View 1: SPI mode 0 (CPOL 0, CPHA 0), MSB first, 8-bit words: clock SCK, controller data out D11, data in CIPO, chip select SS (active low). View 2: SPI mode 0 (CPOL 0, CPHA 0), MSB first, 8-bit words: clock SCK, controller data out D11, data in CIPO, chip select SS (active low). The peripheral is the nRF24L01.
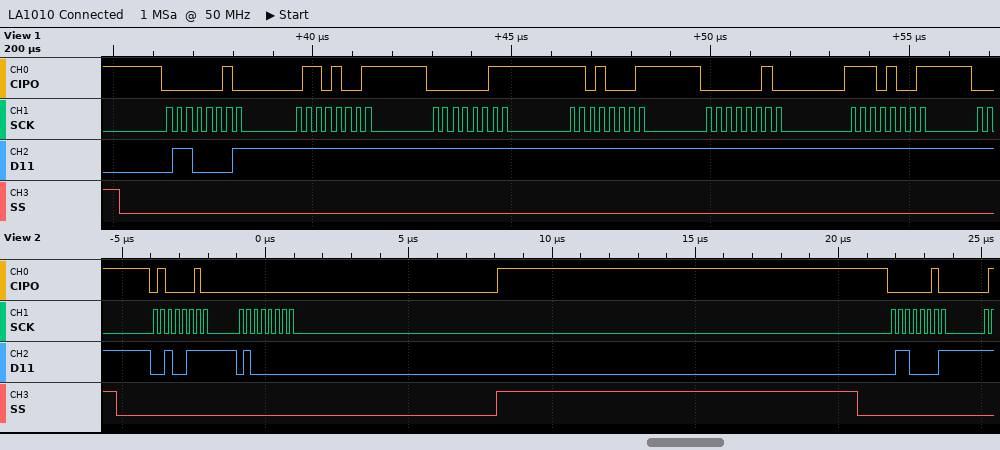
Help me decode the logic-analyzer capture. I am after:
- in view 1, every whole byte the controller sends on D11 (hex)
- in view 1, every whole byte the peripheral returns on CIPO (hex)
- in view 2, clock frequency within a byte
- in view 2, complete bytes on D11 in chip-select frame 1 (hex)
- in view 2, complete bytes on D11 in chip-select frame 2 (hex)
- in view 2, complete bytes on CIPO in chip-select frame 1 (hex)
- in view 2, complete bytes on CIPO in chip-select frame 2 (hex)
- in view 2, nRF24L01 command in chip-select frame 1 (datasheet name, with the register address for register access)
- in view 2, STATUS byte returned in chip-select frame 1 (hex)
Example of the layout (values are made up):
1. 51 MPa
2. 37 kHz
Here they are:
1. 61 FF FF FF FF FF
2. 02 69 03 D1 02 E9
3. 4 MHz
4. 0x27 0x40
5. 0x61
6. 0x42 0x00
7. 0x02
8. W_REGISTER 0x07
9. 0x42
